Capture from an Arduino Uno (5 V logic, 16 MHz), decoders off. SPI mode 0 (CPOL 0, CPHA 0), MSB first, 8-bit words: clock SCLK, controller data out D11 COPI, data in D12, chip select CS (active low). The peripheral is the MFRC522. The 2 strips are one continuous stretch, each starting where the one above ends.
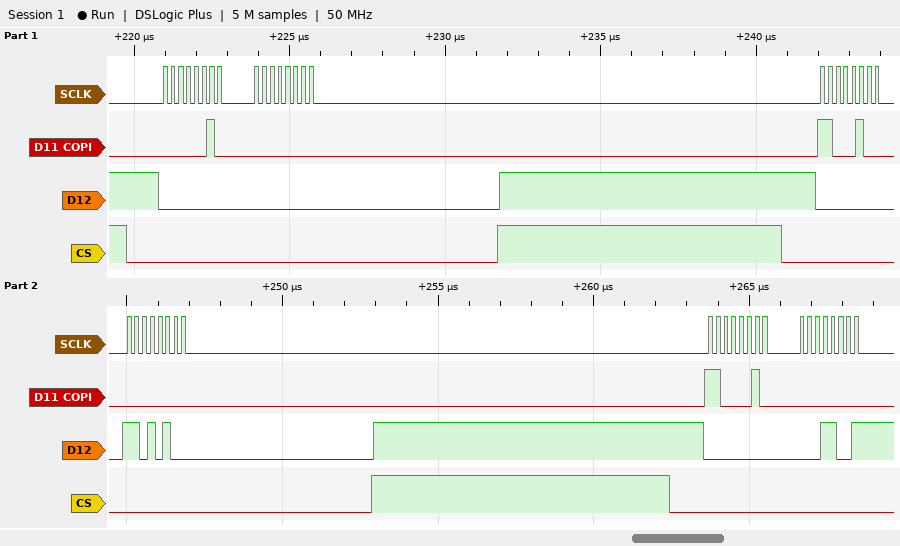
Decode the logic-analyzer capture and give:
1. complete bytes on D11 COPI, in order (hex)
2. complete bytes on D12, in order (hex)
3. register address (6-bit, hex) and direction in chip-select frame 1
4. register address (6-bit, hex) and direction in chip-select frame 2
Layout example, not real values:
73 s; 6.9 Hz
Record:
02 00 C4 00 C2 00; 00 00 00 D4 00 19; 0x01 write; 0x22 read
